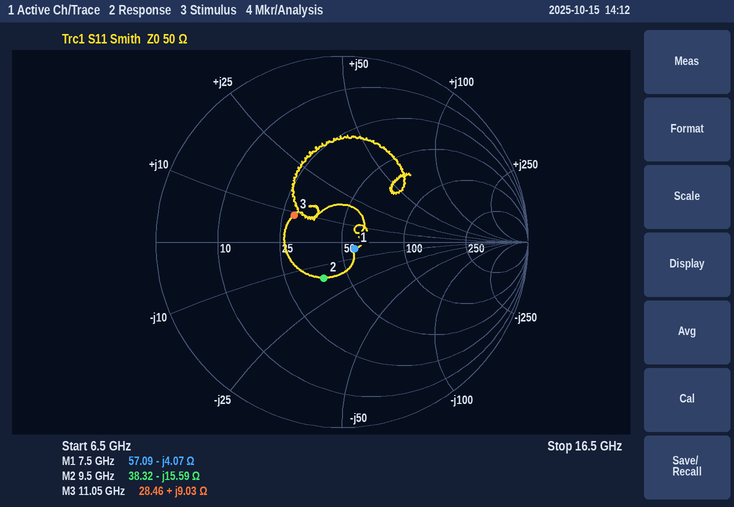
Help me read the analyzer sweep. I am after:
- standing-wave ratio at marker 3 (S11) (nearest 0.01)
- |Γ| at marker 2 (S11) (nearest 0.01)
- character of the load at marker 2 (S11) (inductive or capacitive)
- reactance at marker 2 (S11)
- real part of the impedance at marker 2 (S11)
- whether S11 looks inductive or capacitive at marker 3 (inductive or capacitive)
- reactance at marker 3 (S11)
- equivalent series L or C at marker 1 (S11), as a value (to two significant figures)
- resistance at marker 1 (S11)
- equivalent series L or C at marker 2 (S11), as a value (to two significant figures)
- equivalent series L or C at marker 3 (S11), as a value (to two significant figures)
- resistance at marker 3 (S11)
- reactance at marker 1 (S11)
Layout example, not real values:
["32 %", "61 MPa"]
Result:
["1.84", "0.22", "capacitive", "-15.59 Ω", "38.32 Ω", "inductive", "+9.03 Ω", "5.2 pF", "57.09 Ω", "1.1 pF", "130 pH", "28.46 Ω", "-4.07 Ω"]
